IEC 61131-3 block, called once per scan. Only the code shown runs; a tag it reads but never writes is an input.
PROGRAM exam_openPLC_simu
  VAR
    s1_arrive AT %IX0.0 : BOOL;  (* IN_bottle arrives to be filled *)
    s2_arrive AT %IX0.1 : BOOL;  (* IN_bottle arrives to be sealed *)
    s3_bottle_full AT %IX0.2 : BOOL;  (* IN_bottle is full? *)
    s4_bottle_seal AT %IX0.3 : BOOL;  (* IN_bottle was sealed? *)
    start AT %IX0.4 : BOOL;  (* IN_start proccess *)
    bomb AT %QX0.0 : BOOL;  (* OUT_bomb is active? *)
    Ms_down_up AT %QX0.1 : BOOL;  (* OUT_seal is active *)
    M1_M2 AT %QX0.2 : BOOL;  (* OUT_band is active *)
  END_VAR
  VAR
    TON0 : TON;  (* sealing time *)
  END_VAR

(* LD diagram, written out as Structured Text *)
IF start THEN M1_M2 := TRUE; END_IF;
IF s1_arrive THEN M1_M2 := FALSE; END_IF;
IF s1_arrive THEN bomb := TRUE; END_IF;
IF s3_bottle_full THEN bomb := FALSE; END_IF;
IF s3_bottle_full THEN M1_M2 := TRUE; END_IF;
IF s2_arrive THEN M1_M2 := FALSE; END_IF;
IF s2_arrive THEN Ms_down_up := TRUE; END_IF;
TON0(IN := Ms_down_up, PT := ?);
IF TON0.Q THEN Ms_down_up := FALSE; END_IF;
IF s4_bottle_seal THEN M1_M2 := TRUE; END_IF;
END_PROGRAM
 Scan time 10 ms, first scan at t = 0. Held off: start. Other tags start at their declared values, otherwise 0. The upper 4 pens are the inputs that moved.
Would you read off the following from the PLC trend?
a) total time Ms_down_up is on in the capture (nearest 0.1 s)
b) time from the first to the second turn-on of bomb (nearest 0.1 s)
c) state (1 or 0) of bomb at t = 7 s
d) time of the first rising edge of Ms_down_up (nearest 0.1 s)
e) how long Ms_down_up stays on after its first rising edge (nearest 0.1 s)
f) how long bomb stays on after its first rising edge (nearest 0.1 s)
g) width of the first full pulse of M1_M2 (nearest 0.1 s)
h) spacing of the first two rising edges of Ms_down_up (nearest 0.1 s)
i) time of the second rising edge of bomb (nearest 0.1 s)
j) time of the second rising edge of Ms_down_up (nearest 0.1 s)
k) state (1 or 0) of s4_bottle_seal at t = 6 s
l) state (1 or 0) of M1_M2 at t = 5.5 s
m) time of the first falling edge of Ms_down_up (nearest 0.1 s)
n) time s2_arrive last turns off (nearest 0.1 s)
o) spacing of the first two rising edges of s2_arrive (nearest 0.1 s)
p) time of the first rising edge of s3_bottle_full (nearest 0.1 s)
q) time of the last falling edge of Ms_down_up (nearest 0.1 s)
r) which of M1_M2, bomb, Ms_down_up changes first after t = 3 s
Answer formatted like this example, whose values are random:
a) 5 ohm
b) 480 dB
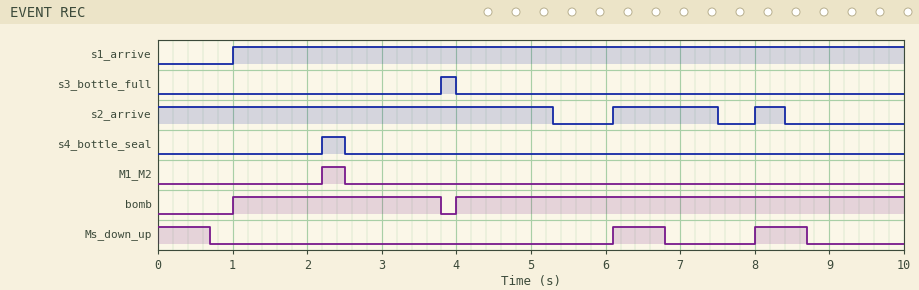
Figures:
a) 2.1 s
b) 3.0 s
c) 1
d) 6.1 s
e) 0.7 s
f) 2.8 s
g) 0.3 s
h) 1.9 s
i) 4.0 s
j) 8.0 s
k) 0
l) 0
m) 0.7 s
n) 8.4 s
o) 1.9 s
p) 3.8 s
q) 8.7 s
r) bomb
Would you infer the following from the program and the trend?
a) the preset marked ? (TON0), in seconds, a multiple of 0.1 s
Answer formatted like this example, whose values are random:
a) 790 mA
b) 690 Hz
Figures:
a) 0.7 s
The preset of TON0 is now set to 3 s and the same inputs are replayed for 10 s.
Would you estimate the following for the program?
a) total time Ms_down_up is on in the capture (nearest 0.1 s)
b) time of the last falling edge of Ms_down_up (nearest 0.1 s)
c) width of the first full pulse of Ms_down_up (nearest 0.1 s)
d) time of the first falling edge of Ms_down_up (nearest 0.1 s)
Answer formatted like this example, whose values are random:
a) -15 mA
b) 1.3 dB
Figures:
a) 6.0 s
b) 9.1 s
c) 3.0 s
d) 3.0 s
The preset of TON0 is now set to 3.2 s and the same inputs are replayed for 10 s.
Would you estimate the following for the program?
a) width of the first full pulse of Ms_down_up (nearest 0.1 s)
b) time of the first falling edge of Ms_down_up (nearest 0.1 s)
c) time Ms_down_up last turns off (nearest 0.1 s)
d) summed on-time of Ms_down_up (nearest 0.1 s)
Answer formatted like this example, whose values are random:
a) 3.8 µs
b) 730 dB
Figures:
a) 3.2 s
b) 3.2 s
c) 9.3 s
d) 6.4 s
